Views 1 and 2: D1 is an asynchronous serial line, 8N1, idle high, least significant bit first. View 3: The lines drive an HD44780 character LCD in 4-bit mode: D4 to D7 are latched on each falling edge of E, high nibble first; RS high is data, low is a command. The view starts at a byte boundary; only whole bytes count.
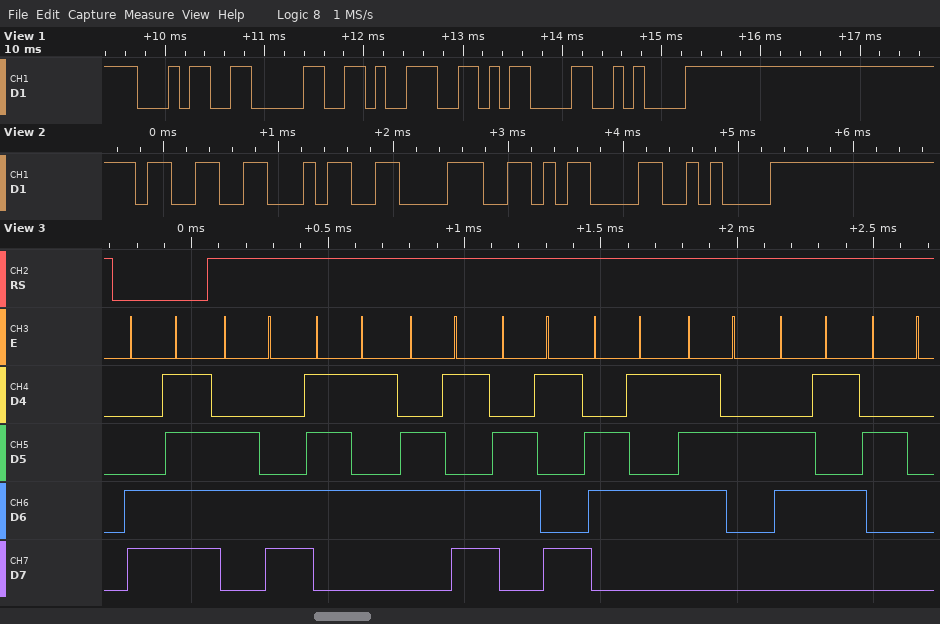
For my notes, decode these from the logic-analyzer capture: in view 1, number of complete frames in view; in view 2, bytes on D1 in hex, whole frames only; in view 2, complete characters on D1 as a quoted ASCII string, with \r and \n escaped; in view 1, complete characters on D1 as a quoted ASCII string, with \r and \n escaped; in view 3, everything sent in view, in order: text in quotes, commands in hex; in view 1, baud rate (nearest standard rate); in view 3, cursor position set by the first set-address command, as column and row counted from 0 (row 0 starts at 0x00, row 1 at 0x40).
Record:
5
0x33 0x34 0x38 0x0D 0x0A
"348\r\n"
"409\r\n"
0xCF "lumiere "
9600 baud
column 15, row 1
